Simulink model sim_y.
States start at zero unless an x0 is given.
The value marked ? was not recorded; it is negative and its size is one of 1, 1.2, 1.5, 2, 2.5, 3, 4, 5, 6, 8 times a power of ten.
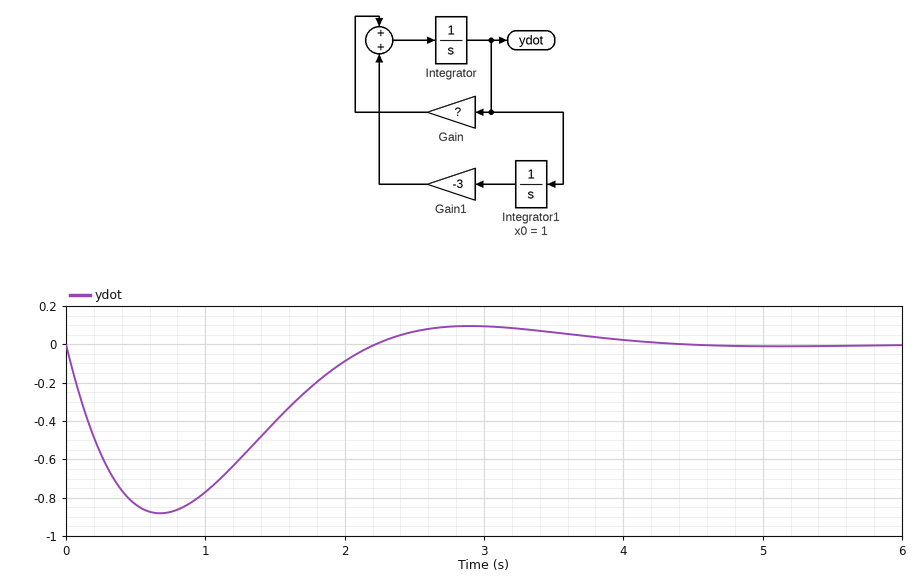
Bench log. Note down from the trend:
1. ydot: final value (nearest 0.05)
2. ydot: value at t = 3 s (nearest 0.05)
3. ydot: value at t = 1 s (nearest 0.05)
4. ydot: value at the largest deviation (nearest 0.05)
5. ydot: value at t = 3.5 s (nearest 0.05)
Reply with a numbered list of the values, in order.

1. 0.00
2. 0.10
3. -0.75
4. -0.90
5. 0.05
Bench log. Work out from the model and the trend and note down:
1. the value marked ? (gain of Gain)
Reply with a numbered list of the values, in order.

1. -2
